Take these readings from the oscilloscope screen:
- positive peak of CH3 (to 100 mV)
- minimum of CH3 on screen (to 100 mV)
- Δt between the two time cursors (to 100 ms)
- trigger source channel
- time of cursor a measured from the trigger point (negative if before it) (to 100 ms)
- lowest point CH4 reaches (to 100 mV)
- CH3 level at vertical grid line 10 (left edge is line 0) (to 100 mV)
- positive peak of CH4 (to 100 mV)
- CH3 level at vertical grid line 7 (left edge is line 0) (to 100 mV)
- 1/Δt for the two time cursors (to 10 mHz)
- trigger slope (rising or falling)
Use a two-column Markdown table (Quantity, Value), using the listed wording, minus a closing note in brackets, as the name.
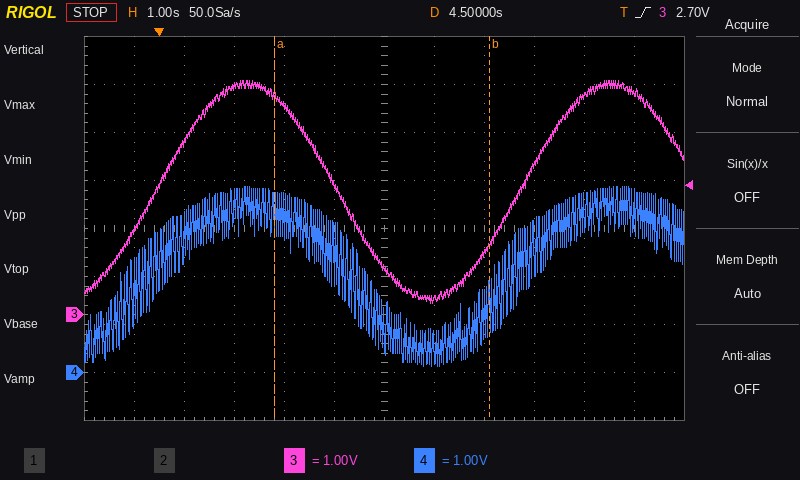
| Quantity | Value |
|---|---|
| positive peak of CH3 | 4.9 V |
| minimum of CH3 on screen | 200 mV |
| Δt between the two time cursors | 4.3 s |
| trigger source channel | CH3 |
| time of cursor a measured from the trigger point (negative if before it) | +2.3 s |
| lowest point CH4 reaches | 100 mV |
| CH3 level at vertical grid line 10 (left edge is line 0) | 4.6 V |
| positive peak of CH4 | 3.9 V |
| CH3 level at vertical grid line 7 (left edge is line 0) | 300 mV |
| 1/Δt for the two time cursors | 230 mHz |
| trigger slope | rising |
